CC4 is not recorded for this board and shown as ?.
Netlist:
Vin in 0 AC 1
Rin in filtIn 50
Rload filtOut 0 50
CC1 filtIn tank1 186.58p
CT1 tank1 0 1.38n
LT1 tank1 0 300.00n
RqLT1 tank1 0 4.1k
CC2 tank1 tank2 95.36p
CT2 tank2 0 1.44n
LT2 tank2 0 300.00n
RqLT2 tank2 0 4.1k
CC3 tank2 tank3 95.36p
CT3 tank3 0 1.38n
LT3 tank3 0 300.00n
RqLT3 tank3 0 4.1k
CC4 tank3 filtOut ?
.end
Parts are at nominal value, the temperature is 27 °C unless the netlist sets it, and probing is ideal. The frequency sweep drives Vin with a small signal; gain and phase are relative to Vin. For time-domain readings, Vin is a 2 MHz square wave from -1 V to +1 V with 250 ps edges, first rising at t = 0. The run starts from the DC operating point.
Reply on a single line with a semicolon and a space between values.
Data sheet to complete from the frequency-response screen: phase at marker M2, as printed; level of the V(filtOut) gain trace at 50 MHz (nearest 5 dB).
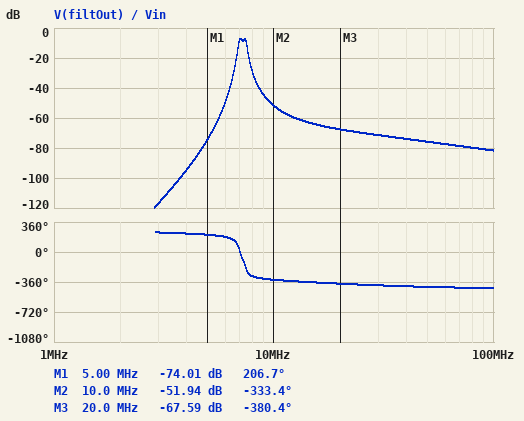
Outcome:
-333.4 deg; -75 dB
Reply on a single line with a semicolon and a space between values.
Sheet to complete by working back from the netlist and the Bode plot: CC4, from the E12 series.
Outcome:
470 pF
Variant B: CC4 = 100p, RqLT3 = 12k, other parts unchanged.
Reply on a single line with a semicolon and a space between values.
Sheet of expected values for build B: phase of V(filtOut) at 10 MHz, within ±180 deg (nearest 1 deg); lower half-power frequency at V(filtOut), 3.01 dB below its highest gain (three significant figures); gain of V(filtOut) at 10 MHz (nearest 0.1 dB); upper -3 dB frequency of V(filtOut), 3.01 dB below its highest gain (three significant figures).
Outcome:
51 deg; 7.16 MHz; -59.8 dB; 7.60 MHz
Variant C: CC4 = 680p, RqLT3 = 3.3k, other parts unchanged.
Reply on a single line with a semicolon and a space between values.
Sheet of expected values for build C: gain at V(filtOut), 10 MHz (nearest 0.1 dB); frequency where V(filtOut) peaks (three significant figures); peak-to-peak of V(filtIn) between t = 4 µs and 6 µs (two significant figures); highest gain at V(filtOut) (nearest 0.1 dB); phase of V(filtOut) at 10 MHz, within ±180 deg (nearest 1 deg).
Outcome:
-51.0 dB; 7.38 MHz; 2.1 V; -7.7 dB; 21 deg
